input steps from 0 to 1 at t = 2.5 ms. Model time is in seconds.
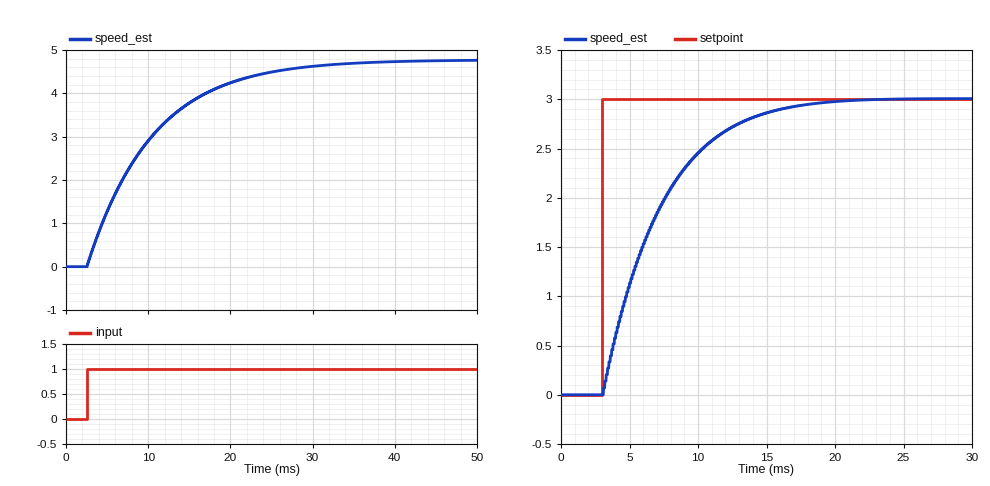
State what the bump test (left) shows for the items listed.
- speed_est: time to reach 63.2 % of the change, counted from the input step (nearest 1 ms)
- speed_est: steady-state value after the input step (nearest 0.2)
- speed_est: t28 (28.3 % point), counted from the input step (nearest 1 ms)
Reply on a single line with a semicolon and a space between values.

8 ms; 4.8; 3 ms
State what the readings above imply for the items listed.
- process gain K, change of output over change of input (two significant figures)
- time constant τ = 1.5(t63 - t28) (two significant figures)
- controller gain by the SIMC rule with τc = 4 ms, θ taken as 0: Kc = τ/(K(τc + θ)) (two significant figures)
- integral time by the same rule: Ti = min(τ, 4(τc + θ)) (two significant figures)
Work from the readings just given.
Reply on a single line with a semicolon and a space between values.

4.8; 7.5 ms; 0.39; 7.5 ms
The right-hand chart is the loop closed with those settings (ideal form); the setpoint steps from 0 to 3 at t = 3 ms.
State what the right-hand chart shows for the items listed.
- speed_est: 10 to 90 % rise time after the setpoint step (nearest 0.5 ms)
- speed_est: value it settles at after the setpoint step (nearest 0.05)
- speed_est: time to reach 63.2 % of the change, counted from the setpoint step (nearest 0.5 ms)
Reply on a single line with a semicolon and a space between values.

9.0 ms; 3.00; 4.0 ms
